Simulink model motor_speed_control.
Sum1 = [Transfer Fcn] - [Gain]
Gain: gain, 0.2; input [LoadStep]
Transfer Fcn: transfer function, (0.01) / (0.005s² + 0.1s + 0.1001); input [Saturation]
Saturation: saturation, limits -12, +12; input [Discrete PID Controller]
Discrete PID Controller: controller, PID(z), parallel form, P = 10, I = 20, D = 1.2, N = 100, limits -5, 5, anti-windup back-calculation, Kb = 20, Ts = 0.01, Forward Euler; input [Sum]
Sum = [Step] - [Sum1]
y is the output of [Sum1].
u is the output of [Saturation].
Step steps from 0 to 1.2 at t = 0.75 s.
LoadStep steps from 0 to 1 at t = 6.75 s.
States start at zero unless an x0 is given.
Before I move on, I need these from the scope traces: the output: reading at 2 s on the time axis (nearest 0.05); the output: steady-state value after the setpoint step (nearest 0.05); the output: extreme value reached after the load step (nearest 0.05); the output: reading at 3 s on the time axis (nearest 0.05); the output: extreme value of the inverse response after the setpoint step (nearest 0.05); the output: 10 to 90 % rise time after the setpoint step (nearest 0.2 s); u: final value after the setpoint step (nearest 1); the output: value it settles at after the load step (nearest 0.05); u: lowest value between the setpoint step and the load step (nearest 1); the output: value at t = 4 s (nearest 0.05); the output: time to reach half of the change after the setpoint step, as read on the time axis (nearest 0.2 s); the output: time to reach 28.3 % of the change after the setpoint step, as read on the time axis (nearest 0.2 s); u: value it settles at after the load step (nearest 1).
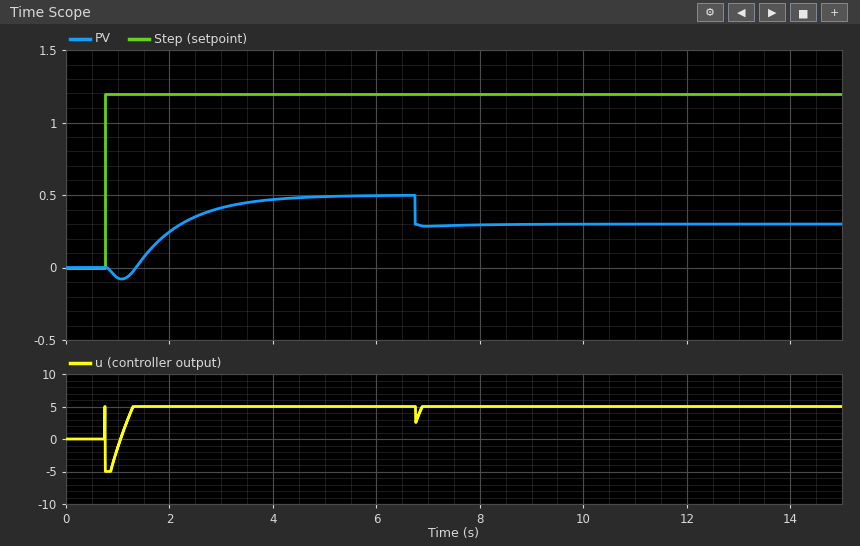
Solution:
0.25
0.50
0.30
0.40
-0.10
2.0 s
5
0.30
-5
0.45
2.0 s
1.6 s
5
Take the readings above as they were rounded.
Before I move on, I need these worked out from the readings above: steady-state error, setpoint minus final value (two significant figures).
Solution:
0.70
